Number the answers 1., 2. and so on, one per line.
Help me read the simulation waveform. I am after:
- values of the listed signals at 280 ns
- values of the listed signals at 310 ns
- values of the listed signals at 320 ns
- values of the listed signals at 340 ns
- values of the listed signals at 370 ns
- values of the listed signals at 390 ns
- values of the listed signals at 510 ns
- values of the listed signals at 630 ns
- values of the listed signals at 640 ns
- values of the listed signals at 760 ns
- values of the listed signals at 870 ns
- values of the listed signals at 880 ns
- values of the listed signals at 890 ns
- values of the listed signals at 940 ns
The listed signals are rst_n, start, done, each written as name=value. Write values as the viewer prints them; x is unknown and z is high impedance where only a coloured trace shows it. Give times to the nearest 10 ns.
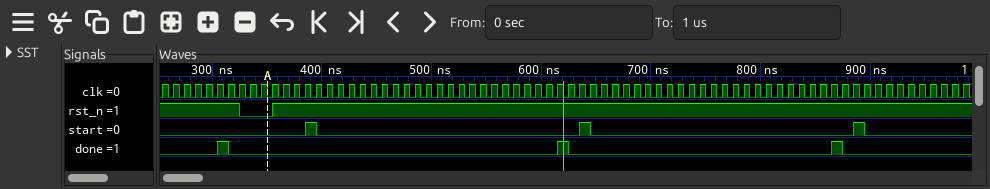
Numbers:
1. rst_n=1, start=0, done=0
2. rst_n=1, start=0, done=1
3. rst_n=1, start=0, done=0
4. rst_n=0, start=0, done=0
5. rst_n=1, start=0, done=0
6. rst_n=1, start=1, done=0
7. rst_n=1, start=0, done=0
8. rst_n=1, start=0, done=0
9. rst_n=1, start=1, done=0
10. rst_n=1, start=0, done=0
11. rst_n=1, start=0, done=1
12. rst_n=1, start=0, done=0
13. rst_n=1, start=1, done=0
14. rst_n=1, start=0, done=0
